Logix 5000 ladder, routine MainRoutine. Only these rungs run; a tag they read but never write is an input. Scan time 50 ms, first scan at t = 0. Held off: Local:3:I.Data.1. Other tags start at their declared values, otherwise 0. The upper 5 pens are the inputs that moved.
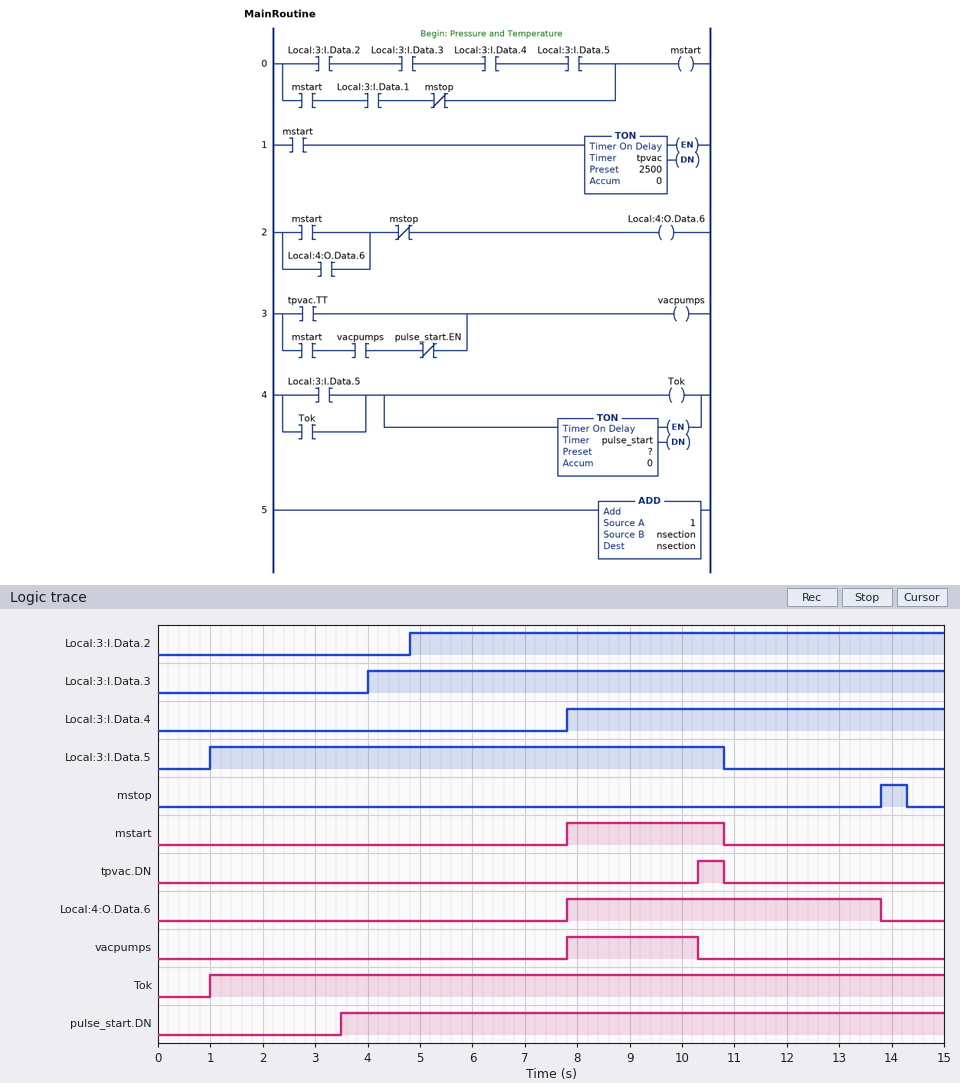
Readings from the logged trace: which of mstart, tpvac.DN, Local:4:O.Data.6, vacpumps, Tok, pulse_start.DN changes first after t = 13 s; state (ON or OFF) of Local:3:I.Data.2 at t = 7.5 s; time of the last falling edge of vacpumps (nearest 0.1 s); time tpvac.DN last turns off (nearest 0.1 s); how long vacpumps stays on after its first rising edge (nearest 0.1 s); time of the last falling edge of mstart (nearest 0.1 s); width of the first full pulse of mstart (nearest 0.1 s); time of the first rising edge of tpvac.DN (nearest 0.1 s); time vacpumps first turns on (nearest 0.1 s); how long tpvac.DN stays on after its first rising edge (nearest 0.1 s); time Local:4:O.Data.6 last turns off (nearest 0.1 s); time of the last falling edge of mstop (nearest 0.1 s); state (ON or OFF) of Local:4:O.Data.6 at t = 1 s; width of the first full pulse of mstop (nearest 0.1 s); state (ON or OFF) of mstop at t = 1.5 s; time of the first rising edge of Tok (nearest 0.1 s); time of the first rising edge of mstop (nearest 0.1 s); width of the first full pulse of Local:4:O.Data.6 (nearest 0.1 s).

Local:4:O.Data.6
ON
10.3 s
10.8 s
2.5 s
10.8 s
3.0 s
10.3 s
7.8 s
0.5 s
13.8 s
14.3 s
OFF
0.5 s
OFF
1.0 s
13.8 s
6.0 s
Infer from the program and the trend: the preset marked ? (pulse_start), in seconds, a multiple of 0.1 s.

2.5 s
